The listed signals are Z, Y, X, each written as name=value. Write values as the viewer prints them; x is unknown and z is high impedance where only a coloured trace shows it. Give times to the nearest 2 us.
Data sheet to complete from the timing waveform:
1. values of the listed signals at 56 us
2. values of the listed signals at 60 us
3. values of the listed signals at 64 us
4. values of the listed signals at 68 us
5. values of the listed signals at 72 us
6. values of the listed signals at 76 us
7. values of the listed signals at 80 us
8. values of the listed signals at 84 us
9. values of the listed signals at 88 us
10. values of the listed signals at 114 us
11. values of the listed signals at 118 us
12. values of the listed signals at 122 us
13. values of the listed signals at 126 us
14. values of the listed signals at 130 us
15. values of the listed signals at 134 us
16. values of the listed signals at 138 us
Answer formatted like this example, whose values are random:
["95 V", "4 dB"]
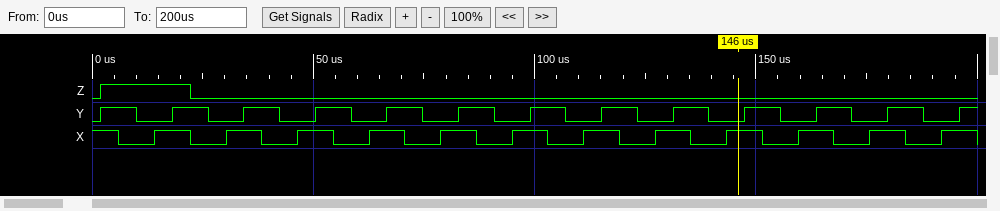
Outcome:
["Z=0, Y=1, X=0", "Z=0, Y=0, X=0", "Z=0, Y=0, X=1", "Z=0, Y=1, X=1", "Z=0, Y=1, X=0", "Z=0, Y=0, X=0", "Z=0, Y=0, X=1", "Z=0, Y=1, X=1", "Z=0, Y=1, X=0", "Z=0, Y=0, X=1", "Z=0, Y=1, X=1", "Z=0, Y=1, X=0", "Z=0, Y=0, X=0", "Z=0, Y=0, X=1", "Z=0, Y=1, X=1", "Z=0, Y=1, X=0"]
